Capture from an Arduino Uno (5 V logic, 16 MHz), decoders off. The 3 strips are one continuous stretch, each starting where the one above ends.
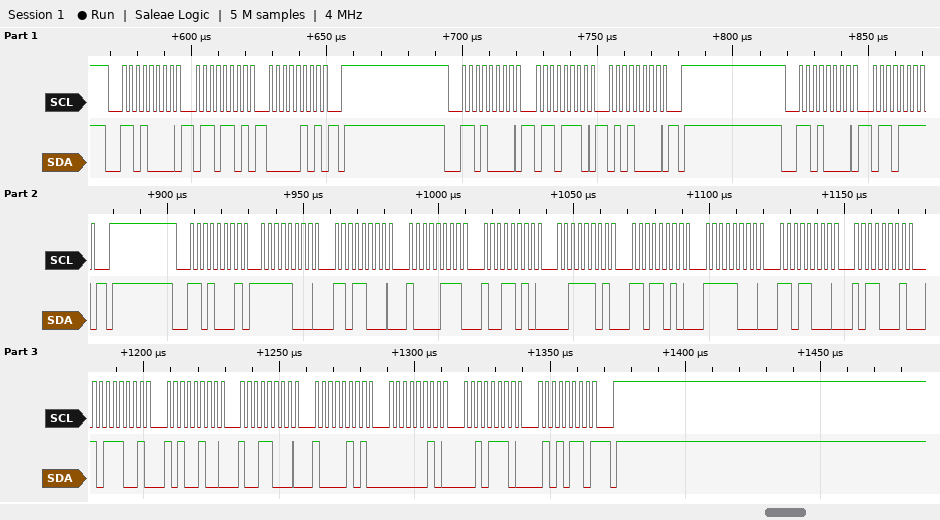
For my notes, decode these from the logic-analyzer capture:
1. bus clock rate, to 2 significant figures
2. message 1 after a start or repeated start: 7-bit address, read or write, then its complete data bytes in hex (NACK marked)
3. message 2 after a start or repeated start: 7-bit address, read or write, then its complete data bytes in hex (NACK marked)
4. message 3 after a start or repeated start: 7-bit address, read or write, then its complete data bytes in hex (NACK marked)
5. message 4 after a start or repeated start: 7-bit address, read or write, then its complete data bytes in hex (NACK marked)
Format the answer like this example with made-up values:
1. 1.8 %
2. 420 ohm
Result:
1. 400 kHz
2. 0x68 write: 6D 05
3. 0x68 write: 6E 50
4. 0x68 write: 6F
5. 0x68 read: F8 D8 87 9A 3D DA F8 D8 B1 B9 A4 98 85 02 2E 56 NACK
